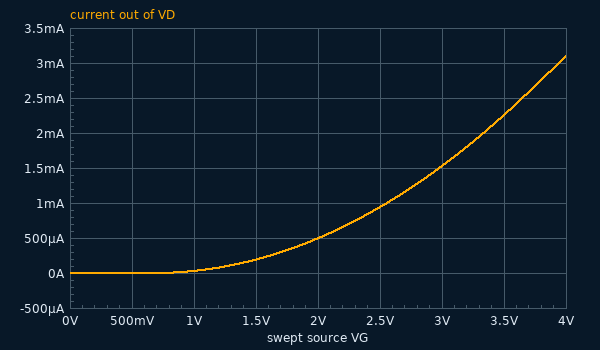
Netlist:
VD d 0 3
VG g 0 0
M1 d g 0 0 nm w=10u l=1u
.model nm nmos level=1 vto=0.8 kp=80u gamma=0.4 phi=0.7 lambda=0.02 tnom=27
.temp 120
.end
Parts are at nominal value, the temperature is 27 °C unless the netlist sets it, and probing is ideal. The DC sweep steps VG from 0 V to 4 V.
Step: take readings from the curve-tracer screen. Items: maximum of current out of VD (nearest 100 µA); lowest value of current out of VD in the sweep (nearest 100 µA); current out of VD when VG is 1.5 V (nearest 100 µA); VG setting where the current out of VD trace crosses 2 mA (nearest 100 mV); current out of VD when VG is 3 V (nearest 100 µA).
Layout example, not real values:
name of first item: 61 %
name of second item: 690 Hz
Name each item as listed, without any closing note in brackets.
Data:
maximum of current out of VD: 3.1 mA
lowest value of current out of VD in the sweep: 0 A
current out of VD when VG is 1.5 V: 200 µA
VG setting where the current out of VD trace crosses 2 mA: 3.3 V
current out of VD when VG is 3 V: 1.5 mA
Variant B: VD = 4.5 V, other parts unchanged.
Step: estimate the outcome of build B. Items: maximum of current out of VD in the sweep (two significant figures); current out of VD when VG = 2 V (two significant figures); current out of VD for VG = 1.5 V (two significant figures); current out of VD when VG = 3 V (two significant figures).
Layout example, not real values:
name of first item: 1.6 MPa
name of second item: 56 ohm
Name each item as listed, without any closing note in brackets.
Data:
maximum of current out of VD in the sweep: 3.2 mA
current out of VD when VG = 2 V: 510 µA
current out of VD for VG = 1.5 V: 200 µA
current out of VD when VG = 3 V: 1.6 mA
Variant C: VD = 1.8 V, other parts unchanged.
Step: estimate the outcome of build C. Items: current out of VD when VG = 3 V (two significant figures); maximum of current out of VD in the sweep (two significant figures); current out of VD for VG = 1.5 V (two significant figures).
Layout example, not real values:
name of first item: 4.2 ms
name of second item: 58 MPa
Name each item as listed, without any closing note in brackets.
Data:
current out of VD when VG = 3 V: 1.4 mA
maximum of current out of VD in the sweep: 2.4 mA
current out of VD for VG = 1.5 V: 190 µA
